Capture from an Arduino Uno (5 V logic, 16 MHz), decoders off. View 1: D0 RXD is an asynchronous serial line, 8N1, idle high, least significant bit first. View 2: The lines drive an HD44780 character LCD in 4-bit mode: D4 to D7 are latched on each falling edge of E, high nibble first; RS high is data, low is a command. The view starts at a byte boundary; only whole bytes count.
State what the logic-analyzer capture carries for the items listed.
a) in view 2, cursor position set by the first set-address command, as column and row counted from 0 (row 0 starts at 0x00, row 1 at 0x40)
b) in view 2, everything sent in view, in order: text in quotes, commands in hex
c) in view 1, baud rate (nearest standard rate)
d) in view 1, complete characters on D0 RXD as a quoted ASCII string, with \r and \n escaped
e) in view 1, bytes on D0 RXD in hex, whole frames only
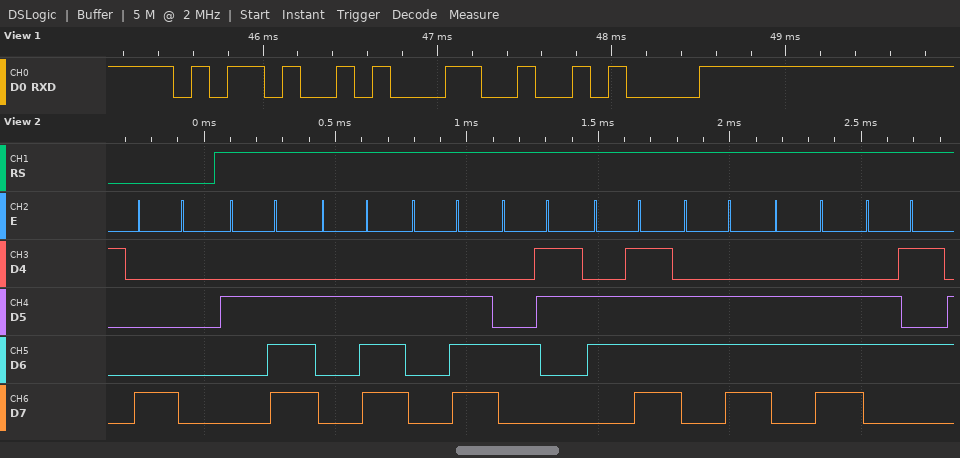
column 0, row 0
0x80 "...Conne"
9600 baud
"-1\n"
2D 31 0A
